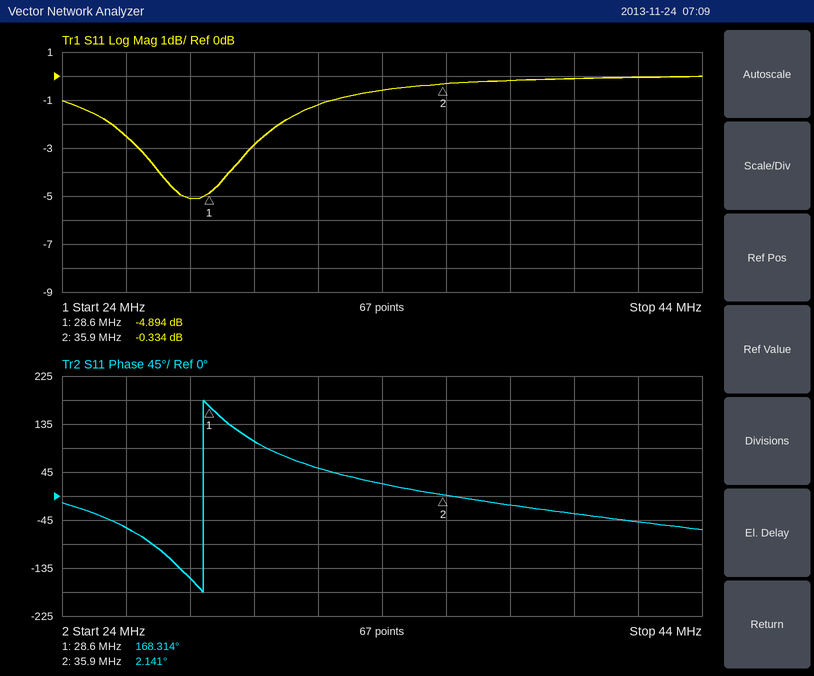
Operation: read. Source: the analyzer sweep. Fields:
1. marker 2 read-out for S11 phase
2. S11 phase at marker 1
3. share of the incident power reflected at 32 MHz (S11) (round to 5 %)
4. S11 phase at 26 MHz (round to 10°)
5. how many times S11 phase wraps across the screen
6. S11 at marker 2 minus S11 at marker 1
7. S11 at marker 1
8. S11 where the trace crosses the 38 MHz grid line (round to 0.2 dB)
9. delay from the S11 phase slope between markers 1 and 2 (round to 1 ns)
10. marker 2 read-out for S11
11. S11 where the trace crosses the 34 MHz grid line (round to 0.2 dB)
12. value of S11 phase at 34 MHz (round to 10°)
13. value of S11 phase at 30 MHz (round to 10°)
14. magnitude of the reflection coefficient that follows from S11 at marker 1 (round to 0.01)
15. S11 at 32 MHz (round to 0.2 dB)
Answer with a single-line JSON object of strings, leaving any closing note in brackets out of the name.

{"marker 2 read-out for S11 phase": "2.141°", "S11 phase at marker 1": "168.314°", "share of the incident power reflected at 32 MHz (S11)": "75 %", "S11 phase at 26 MHz": "-60°", "how many times S11 phase wraps across the screen": "1", "S11 at marker 2 minus S11 at marker 1": "4.560 dB", "S11 at marker 1": "-4.894 dB", "S11 where the trace crosses the 38 MHz grid line": "-0.2 dB", "delay from the S11 phase slope between markers 1 and 2": "63 ns", "marker 2 read-out for S11": "-0.334 dB", "S11 where the trace crosses the 34 MHz grid line": "-0.6 dB", "value of S11 phase at 34 MHz": "20°", "value of S11 phase at 30 MHz": "100°", "magnitude of the reflection coefficient that follows from S11 at marker 1": "0.57", "S11 at 32 MHz": "-1.2 dB"}
